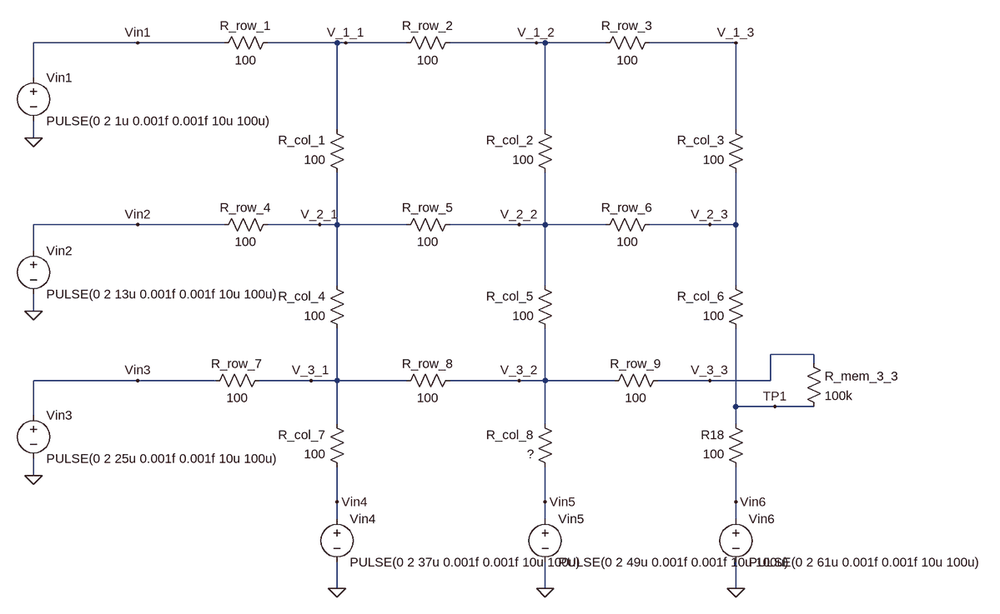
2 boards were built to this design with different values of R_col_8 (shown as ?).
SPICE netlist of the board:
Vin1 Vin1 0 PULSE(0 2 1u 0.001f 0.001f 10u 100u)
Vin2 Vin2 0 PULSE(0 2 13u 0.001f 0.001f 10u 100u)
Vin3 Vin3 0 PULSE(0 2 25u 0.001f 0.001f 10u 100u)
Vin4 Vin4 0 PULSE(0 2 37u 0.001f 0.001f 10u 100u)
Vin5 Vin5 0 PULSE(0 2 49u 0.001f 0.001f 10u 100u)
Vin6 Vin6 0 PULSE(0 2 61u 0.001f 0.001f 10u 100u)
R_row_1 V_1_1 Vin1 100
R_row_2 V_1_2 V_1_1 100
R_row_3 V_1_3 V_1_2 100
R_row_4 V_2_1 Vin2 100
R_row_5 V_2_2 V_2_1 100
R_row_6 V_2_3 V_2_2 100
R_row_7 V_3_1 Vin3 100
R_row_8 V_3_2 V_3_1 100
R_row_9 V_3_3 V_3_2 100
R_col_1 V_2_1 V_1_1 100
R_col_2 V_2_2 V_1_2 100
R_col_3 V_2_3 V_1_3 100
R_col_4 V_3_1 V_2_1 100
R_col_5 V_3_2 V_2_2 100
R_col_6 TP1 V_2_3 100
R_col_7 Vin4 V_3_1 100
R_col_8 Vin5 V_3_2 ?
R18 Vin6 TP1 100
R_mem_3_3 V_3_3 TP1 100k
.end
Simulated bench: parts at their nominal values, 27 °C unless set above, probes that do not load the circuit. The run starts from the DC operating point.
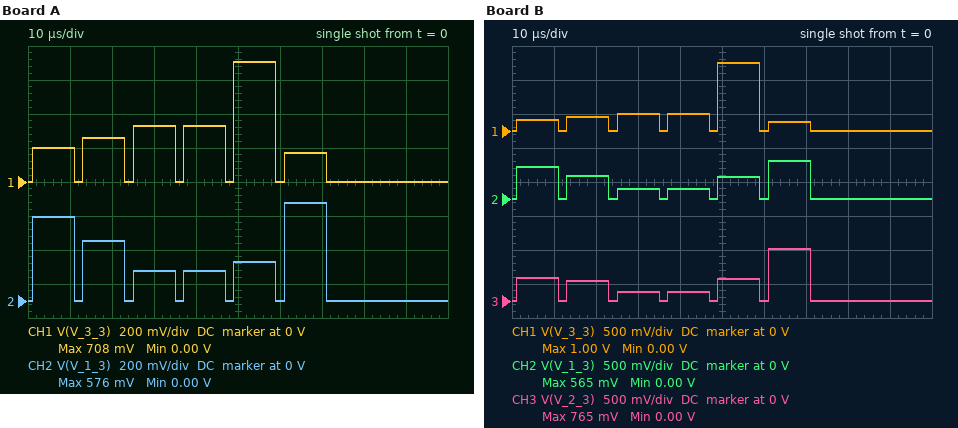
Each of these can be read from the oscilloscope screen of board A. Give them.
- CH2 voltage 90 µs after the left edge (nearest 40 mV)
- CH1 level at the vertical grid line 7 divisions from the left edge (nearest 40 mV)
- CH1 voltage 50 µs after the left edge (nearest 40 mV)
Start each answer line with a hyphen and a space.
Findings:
- 0 V
- 160 mV
- 720 mV
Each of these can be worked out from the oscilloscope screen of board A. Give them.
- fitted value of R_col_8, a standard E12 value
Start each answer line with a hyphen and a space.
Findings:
- 150 Ω
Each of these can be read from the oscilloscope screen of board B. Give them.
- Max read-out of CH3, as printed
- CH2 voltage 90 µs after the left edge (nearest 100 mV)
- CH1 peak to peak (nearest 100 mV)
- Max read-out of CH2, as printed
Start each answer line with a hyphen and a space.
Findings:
- 765 mV
- 0 V
- 1.0 V
- 565 mV
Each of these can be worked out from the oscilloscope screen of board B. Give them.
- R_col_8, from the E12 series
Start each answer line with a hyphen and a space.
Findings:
- 82 Ω
